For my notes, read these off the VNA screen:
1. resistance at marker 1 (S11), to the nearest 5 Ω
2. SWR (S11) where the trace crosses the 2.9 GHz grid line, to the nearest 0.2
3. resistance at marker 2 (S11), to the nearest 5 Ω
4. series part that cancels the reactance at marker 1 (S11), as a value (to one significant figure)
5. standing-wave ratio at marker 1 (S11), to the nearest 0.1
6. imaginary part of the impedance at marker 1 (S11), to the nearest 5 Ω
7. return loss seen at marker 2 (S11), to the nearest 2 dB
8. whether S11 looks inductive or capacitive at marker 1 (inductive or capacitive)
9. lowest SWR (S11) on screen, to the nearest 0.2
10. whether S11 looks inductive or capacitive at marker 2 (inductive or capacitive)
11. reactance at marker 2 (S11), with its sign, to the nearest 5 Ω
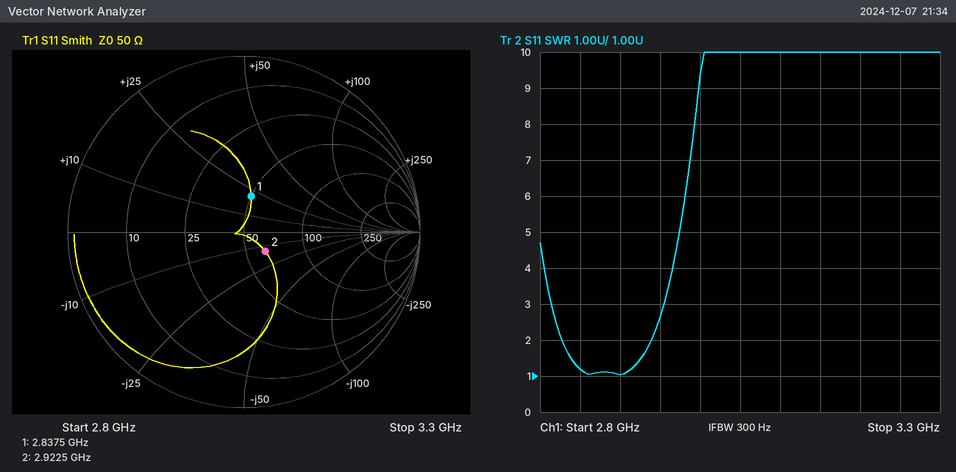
50 Ω
1.0
60 Ω
3 pF
1.5
+20 Ω
16 dB
inductive
1.0
capacitive
-15 Ω
